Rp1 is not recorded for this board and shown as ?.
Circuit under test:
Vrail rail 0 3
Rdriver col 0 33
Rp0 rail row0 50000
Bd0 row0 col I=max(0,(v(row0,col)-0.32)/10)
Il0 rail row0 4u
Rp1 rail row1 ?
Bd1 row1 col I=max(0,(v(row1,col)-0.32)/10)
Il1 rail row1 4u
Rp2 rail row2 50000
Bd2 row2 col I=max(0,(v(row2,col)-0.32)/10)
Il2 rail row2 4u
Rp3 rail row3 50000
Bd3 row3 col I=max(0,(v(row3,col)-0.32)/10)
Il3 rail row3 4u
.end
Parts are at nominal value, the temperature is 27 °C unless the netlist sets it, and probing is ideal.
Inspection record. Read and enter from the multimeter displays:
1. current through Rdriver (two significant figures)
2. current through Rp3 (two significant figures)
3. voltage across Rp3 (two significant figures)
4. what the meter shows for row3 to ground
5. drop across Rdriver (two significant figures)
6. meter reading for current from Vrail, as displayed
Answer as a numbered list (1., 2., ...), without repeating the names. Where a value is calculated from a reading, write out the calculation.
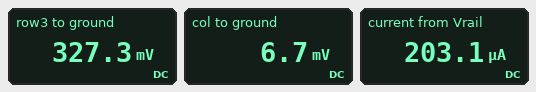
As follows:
1. (6.7 mV) / 33 Ω = 200 µA
2. (3 V - 327.3 mV) / 50 kΩ = 53 µA
3. 3 V - 327.3 mV = 2.7 V
4. 327.3 mV
5. 6.7 mV = 6.7 mV
6. 203.1 µA
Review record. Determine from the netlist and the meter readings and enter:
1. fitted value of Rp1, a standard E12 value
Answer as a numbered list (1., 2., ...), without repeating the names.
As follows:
1. 100 kΩ
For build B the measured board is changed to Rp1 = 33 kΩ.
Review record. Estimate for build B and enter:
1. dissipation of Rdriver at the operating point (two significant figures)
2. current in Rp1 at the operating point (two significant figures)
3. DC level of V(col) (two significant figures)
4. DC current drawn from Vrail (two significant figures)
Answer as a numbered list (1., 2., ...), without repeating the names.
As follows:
1. 2.2 µW
2. 81 µA
3. 8.5 mV
4. 260 µA
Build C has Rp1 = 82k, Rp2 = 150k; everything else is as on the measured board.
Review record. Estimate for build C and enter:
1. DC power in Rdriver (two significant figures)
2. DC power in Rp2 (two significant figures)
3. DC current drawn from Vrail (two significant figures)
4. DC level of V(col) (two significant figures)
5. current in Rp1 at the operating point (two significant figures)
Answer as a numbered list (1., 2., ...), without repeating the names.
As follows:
1. 990 nW
2. 48 µW
3. 170 µA
4. 5.7 mV
5. 33 µA
